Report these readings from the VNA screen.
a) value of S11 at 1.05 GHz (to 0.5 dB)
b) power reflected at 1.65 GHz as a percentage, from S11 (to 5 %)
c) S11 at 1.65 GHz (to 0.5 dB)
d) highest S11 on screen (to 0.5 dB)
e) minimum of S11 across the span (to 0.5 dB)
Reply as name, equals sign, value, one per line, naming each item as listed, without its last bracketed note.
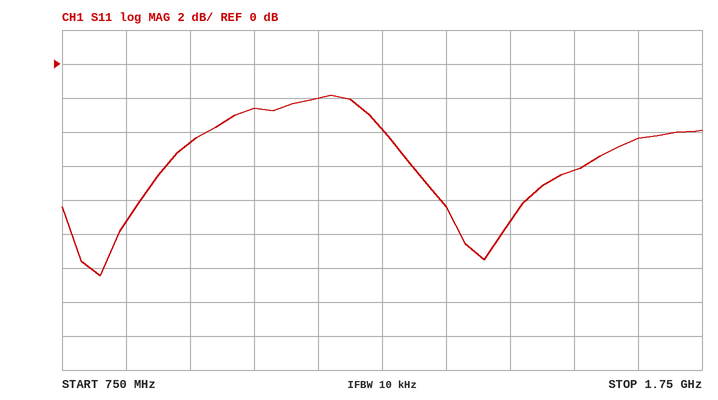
value of S11 at 1.05 GHz = -2.5 dB
power reflected at 1.65 GHz as a percentage, from S11 = 35 %
S11 at 1.65 GHz = -4.5 dB
highest S11 on screen = -2.0 dB
minimum of S11 across the span = -12.5 dB
